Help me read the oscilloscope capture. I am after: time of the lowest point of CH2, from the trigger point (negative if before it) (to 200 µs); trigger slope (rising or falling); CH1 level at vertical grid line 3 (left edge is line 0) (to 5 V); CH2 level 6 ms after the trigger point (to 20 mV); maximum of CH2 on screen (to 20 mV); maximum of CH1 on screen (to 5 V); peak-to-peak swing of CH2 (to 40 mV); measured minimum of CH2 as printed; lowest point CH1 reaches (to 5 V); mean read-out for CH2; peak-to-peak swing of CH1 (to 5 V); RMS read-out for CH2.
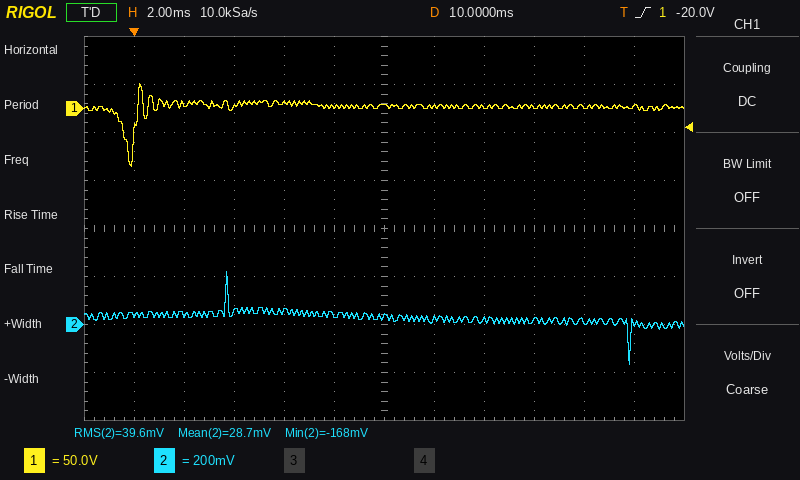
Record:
+19.8 ms
rising
0 V
60 mV
220 mV
25 V
400 mV
-168 mV
-60 V
28.7 mV
85 V
39.6 mV
